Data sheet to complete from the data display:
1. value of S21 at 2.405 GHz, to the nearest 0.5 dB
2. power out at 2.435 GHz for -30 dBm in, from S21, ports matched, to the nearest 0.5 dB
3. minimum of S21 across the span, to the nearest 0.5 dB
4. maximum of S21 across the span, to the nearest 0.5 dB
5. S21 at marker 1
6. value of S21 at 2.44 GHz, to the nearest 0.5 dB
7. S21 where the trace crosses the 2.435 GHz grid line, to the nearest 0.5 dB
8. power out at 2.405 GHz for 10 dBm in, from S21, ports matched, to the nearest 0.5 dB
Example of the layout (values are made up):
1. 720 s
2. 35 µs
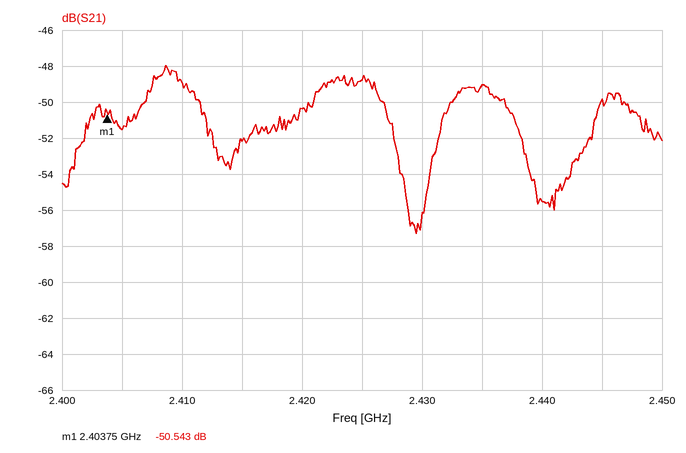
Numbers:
1. -51.5 dB
2. -79.0 dBm
3. -57.5 dB
4. -48.0 dB
5. -50.543 dB
6. -55.5 dB
7. -49.0 dB
8. -41.5 dBm
